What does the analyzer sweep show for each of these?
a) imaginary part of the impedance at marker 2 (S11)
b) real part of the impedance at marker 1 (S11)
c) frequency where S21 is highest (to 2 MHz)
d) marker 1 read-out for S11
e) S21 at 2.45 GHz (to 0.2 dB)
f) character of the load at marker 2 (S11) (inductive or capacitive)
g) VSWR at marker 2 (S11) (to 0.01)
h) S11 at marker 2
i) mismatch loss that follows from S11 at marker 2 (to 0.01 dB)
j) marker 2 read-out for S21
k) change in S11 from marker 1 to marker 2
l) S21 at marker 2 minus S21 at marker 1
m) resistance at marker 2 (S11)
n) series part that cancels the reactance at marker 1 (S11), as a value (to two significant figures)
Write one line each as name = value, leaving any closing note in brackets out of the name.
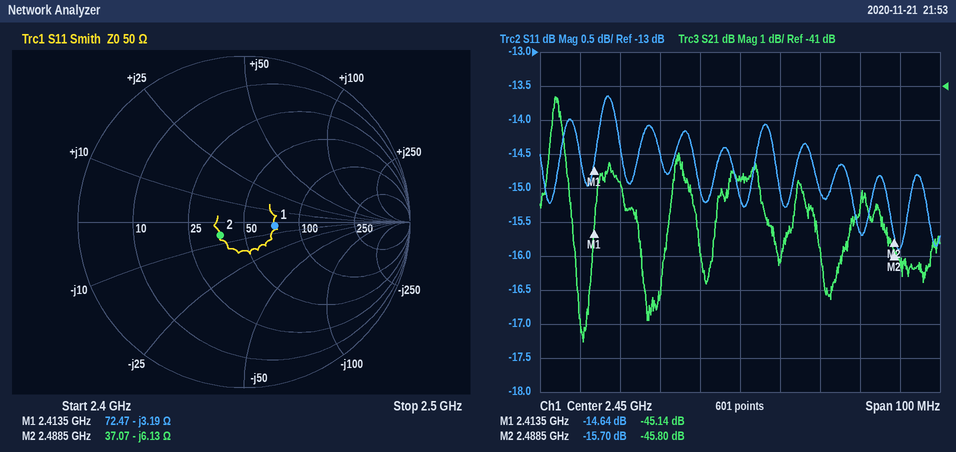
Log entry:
imaginary part of the impedance at marker 2 = -6.13 Ω
real part of the impedance at marker 1 = 72.47 Ω
frequency where S21 is highest = 2.404 GHz
marker 1 read-out for S11 = -14.64 dB
S21 at 2.45 GHz = -43.8 dB
character of the load at marker 2 (S11) = capacitive
VSWR at marker 2 (S11) = 1.39
S11 at marker 2 = -15.70 dB
mismatch loss that follows from S11 at marker 2 = 0.12 dB
marker 2 read-out for S21 = -45.80 dB
change in S11 from marker 1 to marker 2 = -1.06 dB
S21 at marker 2 minus S21 at marker 1 = -0.66 dB
resistance at marker 2 = 37.07 Ω
series part that cancels the reactance at marker 1 (S11), as a value = 210 pH
